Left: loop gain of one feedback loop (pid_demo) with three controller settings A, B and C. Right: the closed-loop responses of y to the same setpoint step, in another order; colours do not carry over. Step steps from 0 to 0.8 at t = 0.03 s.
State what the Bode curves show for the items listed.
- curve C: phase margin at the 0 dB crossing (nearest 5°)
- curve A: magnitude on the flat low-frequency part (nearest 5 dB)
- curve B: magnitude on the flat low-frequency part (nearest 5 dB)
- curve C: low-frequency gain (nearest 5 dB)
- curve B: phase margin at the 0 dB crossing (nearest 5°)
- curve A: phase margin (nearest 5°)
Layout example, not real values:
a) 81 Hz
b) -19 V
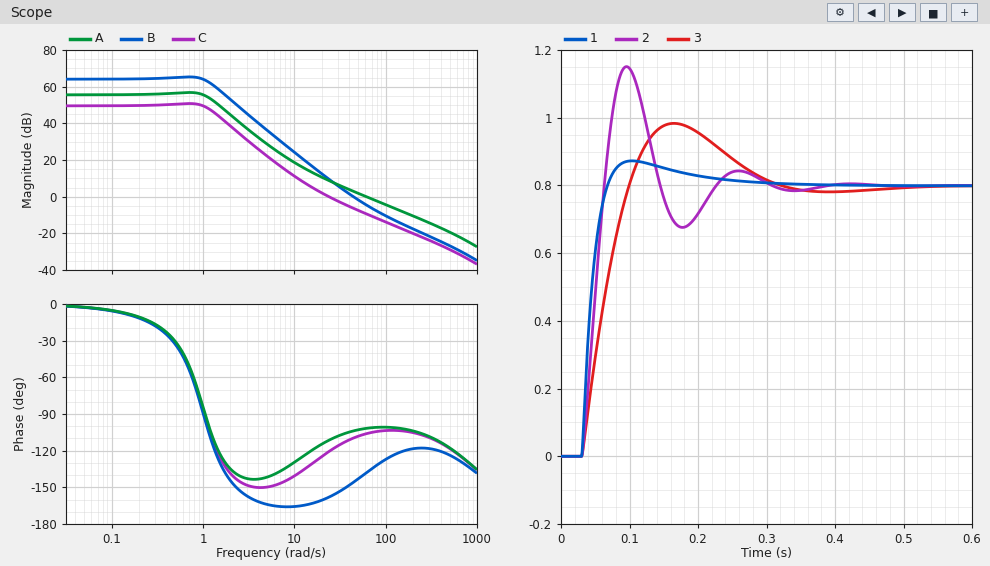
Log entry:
a) 60°
b) 55 dB
c) 65 dB
d) 50 dB
e) 35°
f) 80°
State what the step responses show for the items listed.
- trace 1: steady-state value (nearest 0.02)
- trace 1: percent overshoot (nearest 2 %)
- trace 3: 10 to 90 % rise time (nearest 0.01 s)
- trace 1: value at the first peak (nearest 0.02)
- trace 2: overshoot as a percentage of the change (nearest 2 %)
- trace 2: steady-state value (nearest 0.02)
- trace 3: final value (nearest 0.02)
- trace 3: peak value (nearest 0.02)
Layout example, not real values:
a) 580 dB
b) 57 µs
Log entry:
a) 0.80
b) 10 %
c) 0.05 s
d) 0.88
e) 44 %
f) 0.80
g) 0.80
h) 0.98
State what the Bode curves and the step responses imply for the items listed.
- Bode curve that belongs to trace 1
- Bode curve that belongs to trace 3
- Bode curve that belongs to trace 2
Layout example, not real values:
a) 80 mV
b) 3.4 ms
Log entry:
a) A
b) C
c) B
